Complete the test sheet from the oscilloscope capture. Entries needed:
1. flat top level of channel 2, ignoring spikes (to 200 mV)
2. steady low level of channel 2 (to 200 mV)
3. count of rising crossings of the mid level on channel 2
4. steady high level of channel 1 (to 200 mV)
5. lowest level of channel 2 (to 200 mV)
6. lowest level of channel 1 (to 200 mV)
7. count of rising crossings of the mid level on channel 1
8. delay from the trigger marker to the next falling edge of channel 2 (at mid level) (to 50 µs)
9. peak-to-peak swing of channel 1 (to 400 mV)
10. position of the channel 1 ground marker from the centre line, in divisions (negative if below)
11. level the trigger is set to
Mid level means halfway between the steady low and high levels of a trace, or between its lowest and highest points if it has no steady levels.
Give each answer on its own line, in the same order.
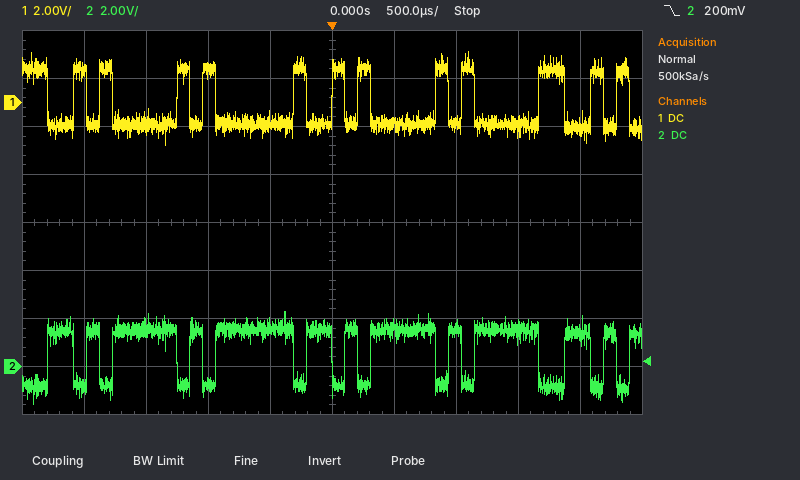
1.6 V
-800 mV
13
1.4 V
-1.6 V
-1.8 V
12
200 µs
4.0 V
+2.5 div
200 mV
